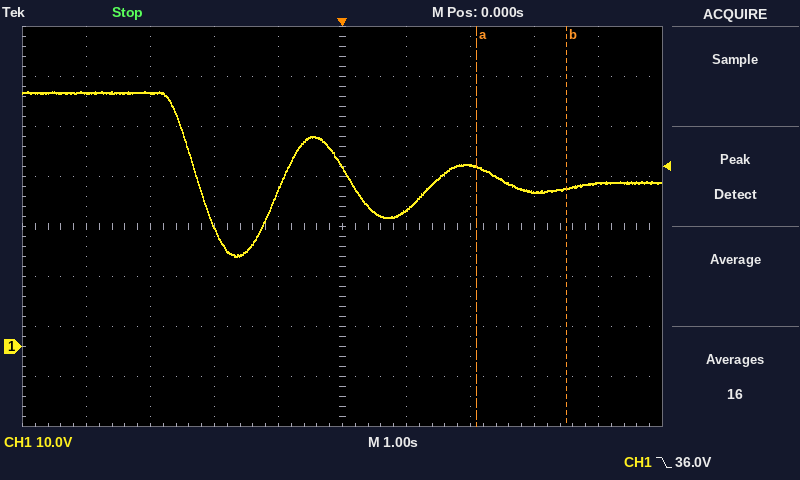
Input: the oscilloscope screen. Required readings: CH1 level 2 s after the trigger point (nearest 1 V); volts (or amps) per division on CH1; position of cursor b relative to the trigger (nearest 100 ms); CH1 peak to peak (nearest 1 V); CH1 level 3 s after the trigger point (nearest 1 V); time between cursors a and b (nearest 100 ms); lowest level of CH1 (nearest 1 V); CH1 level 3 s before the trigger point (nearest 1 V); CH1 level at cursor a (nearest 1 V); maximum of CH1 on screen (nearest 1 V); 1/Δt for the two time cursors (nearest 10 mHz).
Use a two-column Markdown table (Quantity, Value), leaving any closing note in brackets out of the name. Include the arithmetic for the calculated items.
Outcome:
| Quantity | Value |
|---|---|
| CH1 level 2 s after the trigger point | 36 V |
| volts (or amps) per division on CH1 | 10 V |
| position of cursor b relative to the trigger | +3.5 s |
| CH1 peak to peak | 51 V − (18 V) = 33 V |
| CH1 level 3 s after the trigger point | 31 V |
| time between cursors a and b | 1.4 s |
| lowest level of CH1 | 18 V |
| CH1 level 3 s before the trigger point | 51 V |
| CH1 level at cursor a | 36 V |
| maximum of CH1 on screen | 51 V |
| 1/Δt for the two time cursors | 1 / 1.4 s ≈ 710 mHz |
